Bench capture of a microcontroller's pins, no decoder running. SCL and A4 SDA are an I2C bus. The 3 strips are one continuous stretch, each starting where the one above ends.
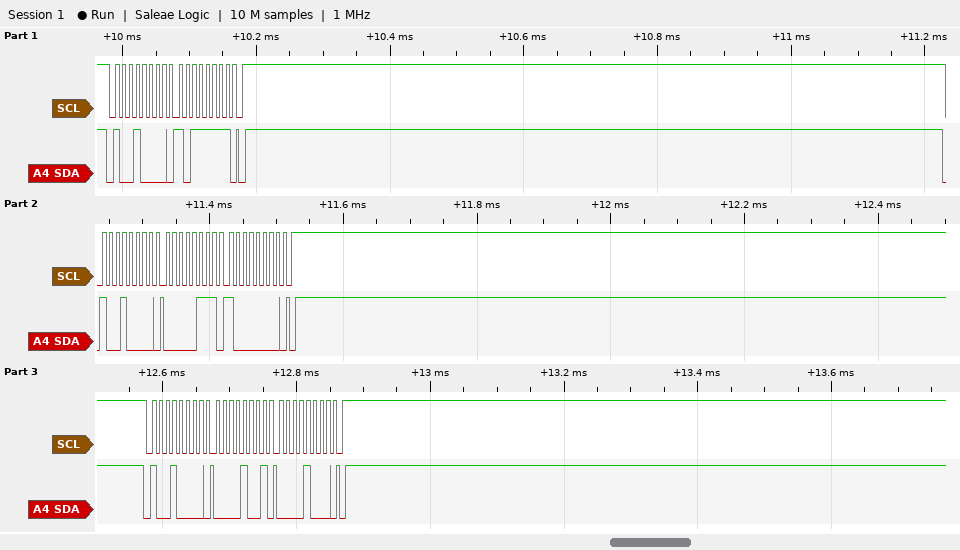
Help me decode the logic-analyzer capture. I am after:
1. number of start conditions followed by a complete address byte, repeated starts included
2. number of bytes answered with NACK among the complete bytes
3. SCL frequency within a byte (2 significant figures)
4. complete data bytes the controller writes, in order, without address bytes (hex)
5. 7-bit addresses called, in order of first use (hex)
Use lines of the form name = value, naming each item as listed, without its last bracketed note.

number of start conditions followed by a complete address byte, repeated starts included = 3
number of bytes answered with NACK among the complete bytes = 0
SCL frequency within a byte = 100 kHz
complete data bytes the controller writes, in order, without address bytes = BF 07 80 09 08
7-bit addresses called, in order of first use = 0x48
